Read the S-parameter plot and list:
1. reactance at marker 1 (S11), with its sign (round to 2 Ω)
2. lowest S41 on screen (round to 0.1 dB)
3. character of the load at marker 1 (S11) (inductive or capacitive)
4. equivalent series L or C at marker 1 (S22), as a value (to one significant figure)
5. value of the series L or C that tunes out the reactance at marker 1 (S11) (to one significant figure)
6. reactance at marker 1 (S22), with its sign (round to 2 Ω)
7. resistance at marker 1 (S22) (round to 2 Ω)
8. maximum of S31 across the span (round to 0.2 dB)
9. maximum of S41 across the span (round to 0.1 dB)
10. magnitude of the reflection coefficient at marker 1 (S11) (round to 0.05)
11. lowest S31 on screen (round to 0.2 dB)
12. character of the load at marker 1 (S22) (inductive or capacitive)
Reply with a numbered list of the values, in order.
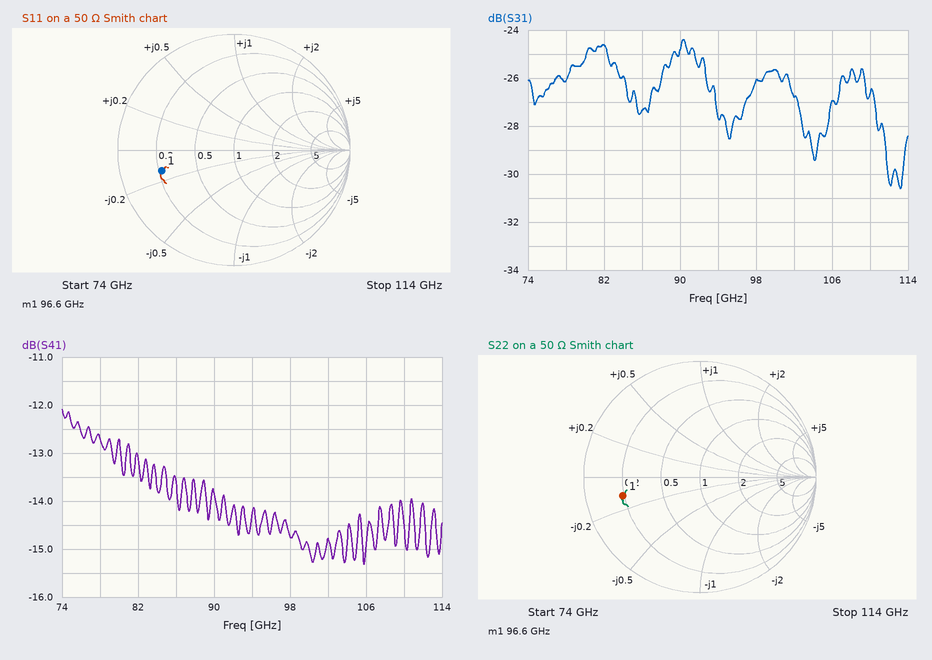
1. -6 Ω
2. -15.3 dB
3. capacitive
4. 300 fF
5. 10 pH
6. -6 Ω
7. 10 Ω
8. -24.4 dB
9. -12.1 dB
10. 0.65
11. -30.6 dB
12. capacitive
